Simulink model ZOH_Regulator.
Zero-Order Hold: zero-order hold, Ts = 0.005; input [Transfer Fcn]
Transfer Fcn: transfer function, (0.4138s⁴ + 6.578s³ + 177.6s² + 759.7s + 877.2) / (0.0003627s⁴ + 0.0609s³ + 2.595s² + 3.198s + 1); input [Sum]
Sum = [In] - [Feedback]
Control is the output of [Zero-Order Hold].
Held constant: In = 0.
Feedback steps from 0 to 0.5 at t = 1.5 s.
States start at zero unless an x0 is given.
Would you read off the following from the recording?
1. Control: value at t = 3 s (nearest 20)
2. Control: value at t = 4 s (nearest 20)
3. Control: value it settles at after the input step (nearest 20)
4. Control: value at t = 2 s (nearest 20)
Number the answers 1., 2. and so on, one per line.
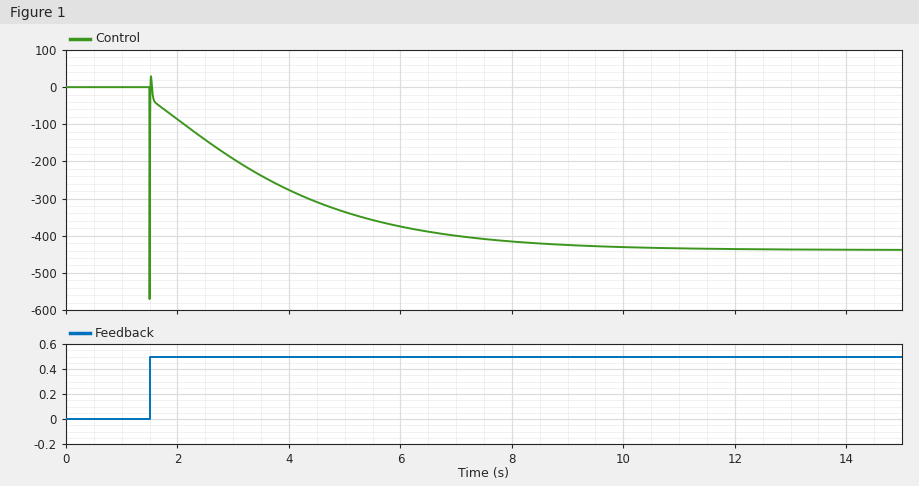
1. -200
2. -280
3. -440
4. -80
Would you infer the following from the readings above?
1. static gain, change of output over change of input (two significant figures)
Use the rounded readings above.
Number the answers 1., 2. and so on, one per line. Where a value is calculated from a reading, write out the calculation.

1. (-440 - 0) / (0.5 - 0) = -880
